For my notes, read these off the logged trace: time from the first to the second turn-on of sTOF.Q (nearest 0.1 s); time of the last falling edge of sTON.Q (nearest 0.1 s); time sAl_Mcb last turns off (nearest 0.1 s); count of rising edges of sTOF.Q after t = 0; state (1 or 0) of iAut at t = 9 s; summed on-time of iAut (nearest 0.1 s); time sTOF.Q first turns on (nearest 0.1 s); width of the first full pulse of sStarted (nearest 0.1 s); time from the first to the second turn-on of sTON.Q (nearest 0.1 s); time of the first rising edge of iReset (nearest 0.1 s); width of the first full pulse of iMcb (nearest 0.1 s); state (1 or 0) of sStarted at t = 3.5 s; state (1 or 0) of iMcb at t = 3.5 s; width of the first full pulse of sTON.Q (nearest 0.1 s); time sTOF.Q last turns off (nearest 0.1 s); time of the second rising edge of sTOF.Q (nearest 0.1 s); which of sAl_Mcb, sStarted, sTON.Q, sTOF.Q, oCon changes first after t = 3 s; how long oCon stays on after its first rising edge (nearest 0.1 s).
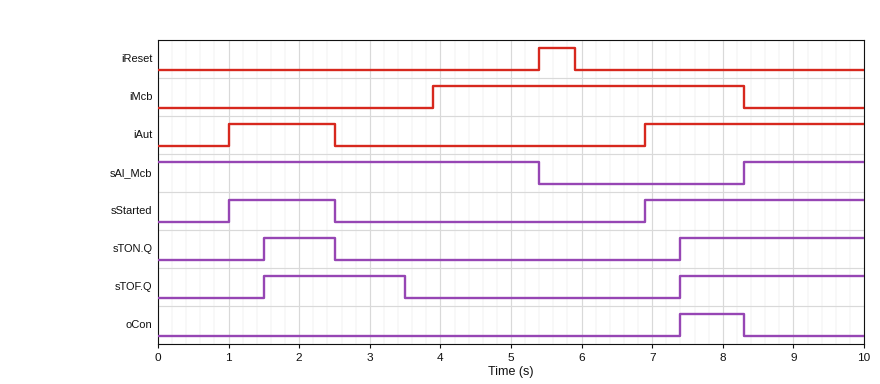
5.9 s
2.5 s
5.4 s
2
1
4.6 s
1.5 s
1.5 s
5.9 s
5.4 s
4.4 s
0
0
1.0 s
3.5 s
7.4 s
sTOF.Q
0.9 s
